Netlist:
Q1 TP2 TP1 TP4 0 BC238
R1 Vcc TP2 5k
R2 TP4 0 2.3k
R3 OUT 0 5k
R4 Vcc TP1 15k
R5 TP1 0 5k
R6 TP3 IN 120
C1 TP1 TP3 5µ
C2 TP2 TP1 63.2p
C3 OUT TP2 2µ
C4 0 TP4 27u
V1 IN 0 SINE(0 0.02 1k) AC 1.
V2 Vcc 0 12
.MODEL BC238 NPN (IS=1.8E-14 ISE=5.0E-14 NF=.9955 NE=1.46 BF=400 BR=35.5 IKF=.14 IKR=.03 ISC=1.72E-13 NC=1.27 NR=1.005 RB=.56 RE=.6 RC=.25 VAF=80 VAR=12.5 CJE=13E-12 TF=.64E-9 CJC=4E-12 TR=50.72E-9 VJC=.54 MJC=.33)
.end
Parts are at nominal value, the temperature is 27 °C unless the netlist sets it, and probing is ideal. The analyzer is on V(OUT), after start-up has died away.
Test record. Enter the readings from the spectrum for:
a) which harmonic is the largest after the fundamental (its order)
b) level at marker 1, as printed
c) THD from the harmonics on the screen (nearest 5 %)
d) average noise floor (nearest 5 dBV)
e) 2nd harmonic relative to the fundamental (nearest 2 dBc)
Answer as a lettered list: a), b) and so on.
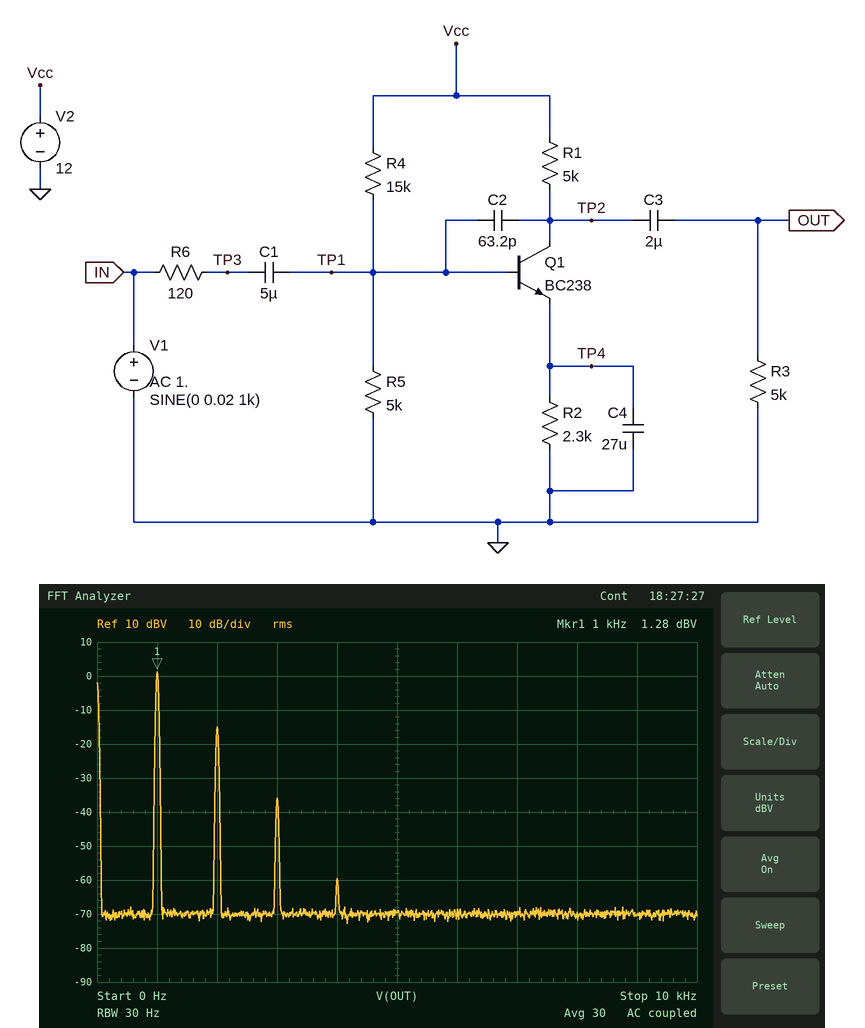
a) 2
b) 1.28 dBV
c) 15 %
d) -70 dBV
e) -16 dBc
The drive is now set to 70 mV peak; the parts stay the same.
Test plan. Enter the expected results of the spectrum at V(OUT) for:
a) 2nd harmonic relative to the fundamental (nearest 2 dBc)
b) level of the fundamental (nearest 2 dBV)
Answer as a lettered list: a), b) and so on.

a) -8 dBc
b) 8 dBV
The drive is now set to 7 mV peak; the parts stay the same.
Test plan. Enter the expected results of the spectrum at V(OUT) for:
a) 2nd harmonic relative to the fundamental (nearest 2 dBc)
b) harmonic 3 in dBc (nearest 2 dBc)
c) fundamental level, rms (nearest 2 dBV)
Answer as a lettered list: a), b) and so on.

a) -26 dBc
b) -56 dBc
c) -8 dBV
